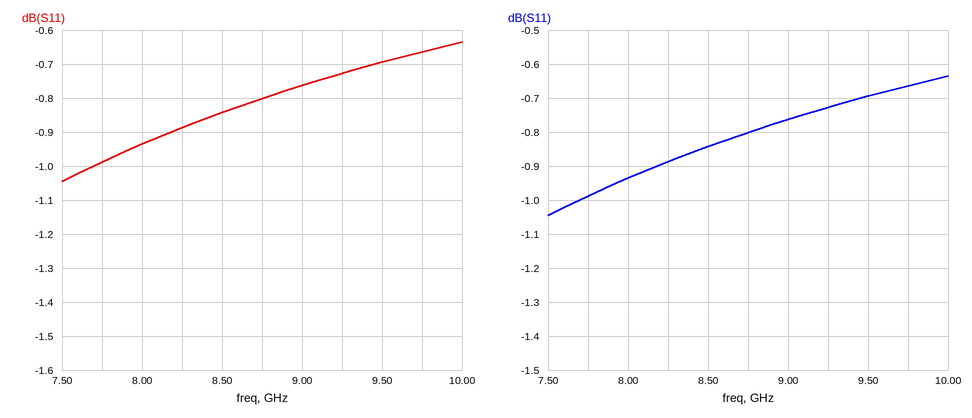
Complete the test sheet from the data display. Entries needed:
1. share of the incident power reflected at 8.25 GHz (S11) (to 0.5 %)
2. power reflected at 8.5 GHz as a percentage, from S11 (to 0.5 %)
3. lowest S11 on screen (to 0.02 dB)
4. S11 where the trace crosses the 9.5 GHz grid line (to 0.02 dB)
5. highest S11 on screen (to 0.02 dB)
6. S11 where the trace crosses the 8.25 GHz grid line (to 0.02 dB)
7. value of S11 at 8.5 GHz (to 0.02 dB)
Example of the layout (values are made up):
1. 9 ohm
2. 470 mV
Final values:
1. 81.5 %
2. 82.5 %
3. -1.04 dB
4. -0.70 dB
5. -0.64 dB
6. -0.88 dB
7. -0.84 dB
